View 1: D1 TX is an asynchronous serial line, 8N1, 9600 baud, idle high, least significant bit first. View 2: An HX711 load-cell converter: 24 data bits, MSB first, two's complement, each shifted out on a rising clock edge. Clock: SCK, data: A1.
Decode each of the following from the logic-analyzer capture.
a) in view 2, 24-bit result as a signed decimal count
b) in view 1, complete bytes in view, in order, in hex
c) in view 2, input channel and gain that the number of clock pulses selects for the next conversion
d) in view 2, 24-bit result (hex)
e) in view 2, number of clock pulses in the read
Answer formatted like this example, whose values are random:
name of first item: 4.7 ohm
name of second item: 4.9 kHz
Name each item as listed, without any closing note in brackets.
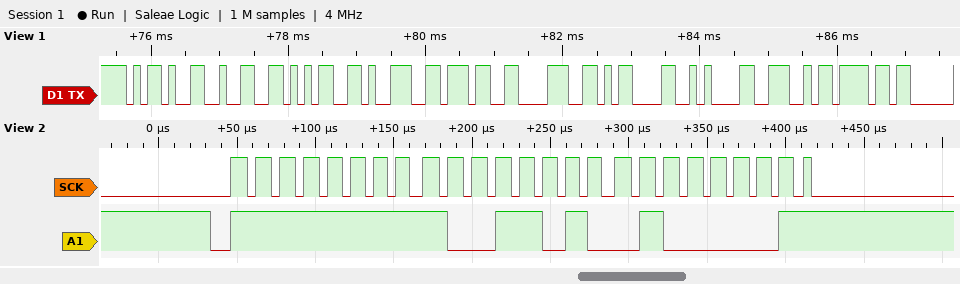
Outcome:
in view 2, 24-bit result as a signed decimal count: -26047
in view 1, complete bytes in view, in order, in hex: 2D 32 35 39 37 38 0D 0A 4E 6F
in view 2, input channel and gain that the number of clock pulses selects for the next conversion: channel A, gain 128
in view 2, 24-bit result: 0xFF9A41
in view 2, number of clock pulses in the read: 25
